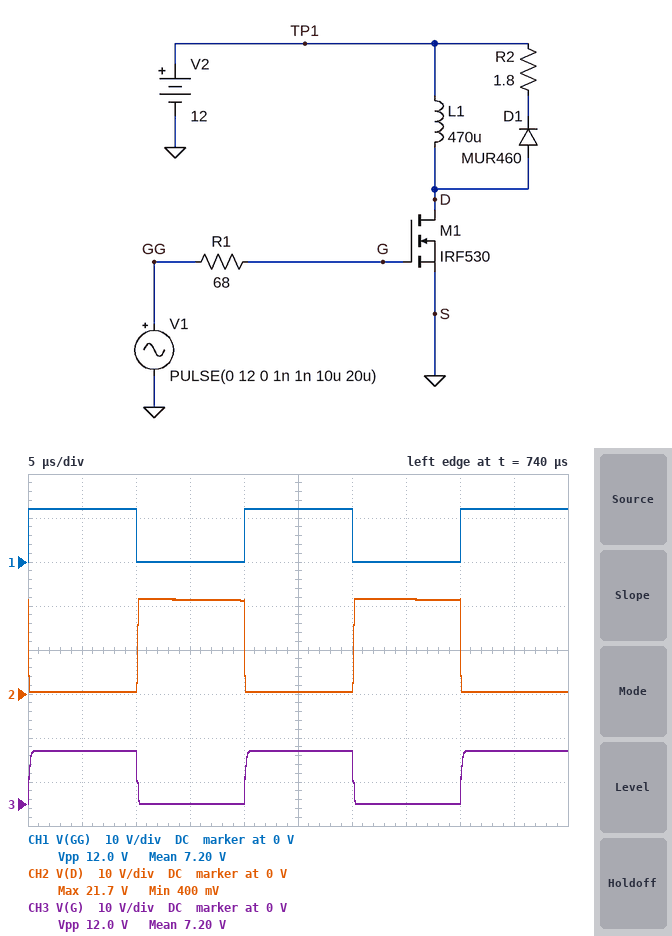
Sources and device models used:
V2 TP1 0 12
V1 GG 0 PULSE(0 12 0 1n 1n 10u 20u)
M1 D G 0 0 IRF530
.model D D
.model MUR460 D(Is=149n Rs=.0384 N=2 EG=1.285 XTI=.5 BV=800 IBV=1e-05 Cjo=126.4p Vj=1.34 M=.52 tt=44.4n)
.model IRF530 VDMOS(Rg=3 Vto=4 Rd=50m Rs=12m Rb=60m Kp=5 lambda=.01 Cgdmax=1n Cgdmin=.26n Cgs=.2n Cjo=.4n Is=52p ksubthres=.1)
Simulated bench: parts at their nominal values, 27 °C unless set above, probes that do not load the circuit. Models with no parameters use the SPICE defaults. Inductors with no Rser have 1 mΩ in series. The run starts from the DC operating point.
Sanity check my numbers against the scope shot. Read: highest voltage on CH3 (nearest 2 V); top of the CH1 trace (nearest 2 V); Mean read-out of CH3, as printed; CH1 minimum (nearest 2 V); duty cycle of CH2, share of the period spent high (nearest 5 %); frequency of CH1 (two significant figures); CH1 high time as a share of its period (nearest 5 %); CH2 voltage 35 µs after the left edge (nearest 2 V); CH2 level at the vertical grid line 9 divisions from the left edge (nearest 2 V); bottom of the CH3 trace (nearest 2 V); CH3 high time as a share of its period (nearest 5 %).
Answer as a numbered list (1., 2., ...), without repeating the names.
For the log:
1. 12 V
2. 12 V
3. 7.20 V
4. 0 V
5. 50 %
6. 50 kHz
7. 50 %
8. 22 V
9. 0 V
10. 0 V
11. 50 %
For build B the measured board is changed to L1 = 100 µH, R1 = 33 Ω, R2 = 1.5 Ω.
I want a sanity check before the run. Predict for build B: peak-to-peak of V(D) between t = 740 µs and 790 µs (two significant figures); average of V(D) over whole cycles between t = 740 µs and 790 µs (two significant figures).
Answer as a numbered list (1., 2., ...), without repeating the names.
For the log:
1. 24 V
2. 12 V
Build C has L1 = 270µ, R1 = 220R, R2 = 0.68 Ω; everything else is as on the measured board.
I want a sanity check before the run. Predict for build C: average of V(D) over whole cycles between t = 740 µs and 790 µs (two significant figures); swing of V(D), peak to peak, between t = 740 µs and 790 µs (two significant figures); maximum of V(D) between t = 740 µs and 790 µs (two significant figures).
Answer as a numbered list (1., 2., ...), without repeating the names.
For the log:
1. 10 V
2. 19 V
3. 20 V
